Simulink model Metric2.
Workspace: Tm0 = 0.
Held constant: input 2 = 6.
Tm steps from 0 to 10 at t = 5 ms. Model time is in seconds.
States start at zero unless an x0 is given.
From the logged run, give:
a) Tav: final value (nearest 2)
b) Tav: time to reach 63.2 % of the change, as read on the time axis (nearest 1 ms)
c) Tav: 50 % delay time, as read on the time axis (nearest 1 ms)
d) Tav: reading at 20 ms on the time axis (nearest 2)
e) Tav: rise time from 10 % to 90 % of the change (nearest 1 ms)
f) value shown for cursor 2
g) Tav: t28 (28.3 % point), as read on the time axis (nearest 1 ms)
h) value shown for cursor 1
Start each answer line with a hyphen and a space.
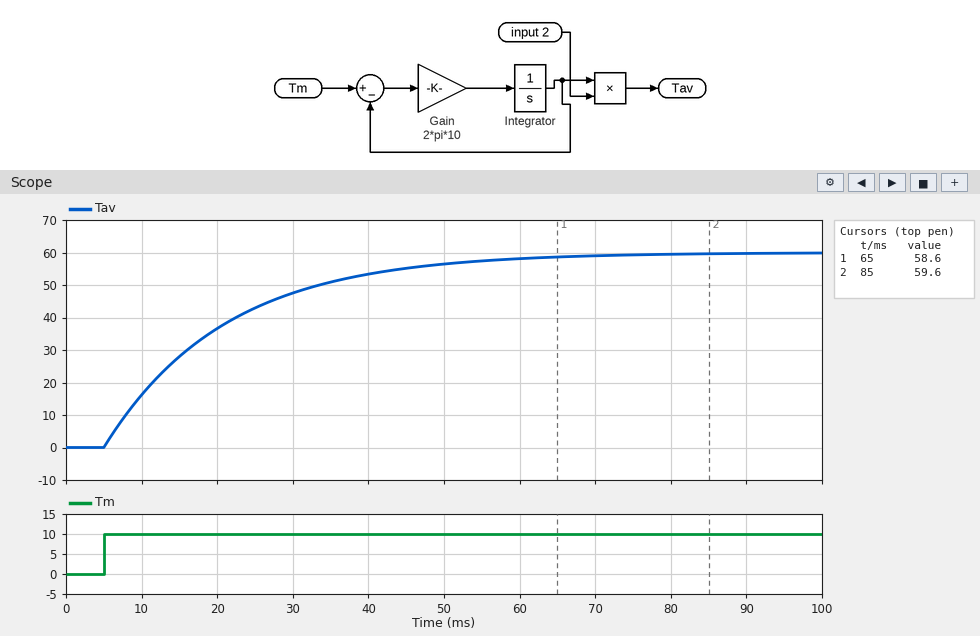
- 60
- 21 ms
- 16 ms
- 36
- 35 ms
- 59.6
- 10 ms
- 58.6
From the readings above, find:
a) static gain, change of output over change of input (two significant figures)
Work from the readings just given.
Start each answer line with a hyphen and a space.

- 6.0
